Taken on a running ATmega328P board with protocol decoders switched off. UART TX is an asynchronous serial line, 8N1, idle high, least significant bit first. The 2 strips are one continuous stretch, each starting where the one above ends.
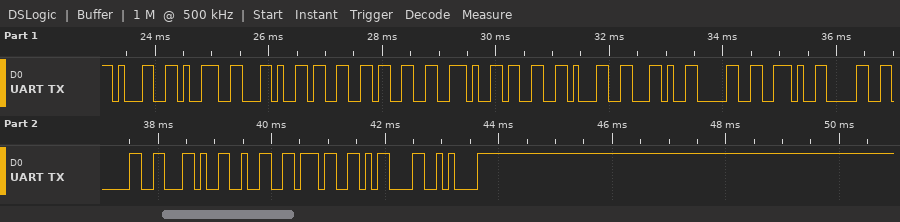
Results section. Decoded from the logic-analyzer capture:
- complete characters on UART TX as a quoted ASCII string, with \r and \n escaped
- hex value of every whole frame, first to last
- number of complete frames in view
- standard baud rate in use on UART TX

"19,33.31,0.00,27\r\n"
31 39 2C 33 33 2E 33 31 2C 30 2E 30 30 2C 32 37 0D 0A
18
9600 baud
